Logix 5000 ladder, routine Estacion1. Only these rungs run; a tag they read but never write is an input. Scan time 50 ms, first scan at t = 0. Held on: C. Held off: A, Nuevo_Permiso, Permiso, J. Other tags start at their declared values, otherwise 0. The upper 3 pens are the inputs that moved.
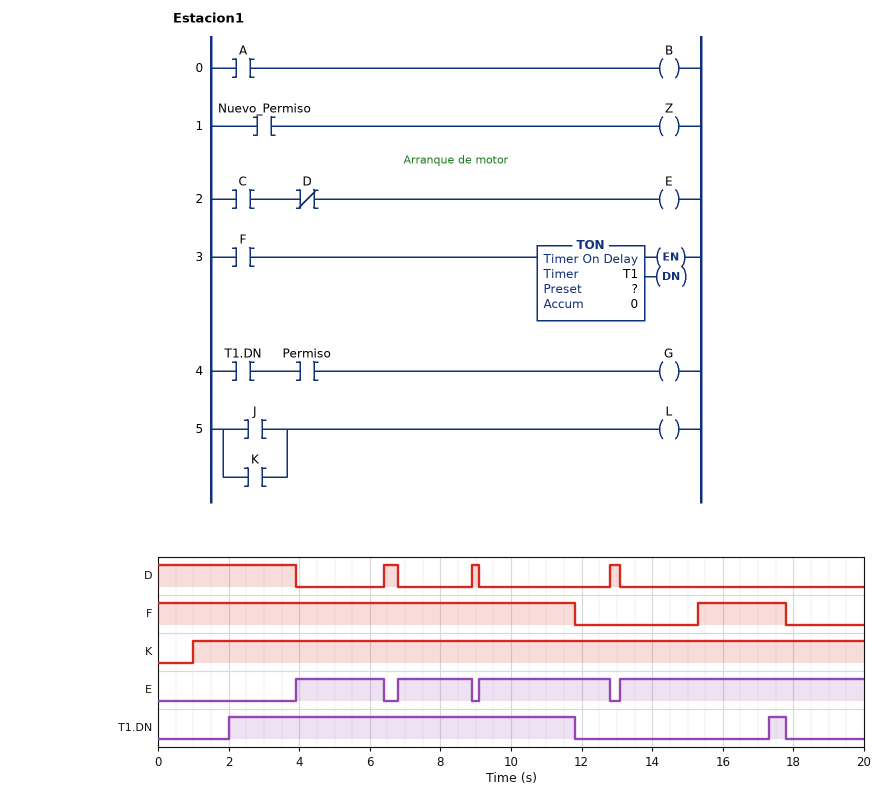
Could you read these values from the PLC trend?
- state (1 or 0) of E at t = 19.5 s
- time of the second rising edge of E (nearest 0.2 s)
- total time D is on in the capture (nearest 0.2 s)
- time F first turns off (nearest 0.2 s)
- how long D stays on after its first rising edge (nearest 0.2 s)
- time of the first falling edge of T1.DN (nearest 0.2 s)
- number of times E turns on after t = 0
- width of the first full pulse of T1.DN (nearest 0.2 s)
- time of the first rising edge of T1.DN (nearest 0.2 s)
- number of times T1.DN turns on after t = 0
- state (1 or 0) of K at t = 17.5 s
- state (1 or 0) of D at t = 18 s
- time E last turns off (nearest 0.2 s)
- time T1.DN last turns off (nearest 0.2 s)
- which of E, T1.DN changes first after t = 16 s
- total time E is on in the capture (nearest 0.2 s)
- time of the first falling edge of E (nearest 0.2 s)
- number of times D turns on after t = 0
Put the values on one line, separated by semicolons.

1; 6.8 s; 4.8 s; 11.8 s; 0.4 s; 11.8 s; 4; 9.8 s; 2.0 s; 2; 1; 0; 12.8 s; 17.8 s; T1.DN; 15.2 s; 6.4 s; 3
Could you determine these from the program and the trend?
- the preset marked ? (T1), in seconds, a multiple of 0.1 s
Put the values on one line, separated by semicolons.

2.0 s
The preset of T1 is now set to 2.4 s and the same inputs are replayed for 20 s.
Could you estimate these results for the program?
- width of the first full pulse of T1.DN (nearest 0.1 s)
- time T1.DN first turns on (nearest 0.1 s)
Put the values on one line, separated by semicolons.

9.4 s; 2.4 s
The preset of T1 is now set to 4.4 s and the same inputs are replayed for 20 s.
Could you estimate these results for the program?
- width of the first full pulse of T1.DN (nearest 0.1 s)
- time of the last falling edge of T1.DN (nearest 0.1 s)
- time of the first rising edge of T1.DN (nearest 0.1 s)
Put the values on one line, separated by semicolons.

7.4 s; 11.8 s; 4.4 s
